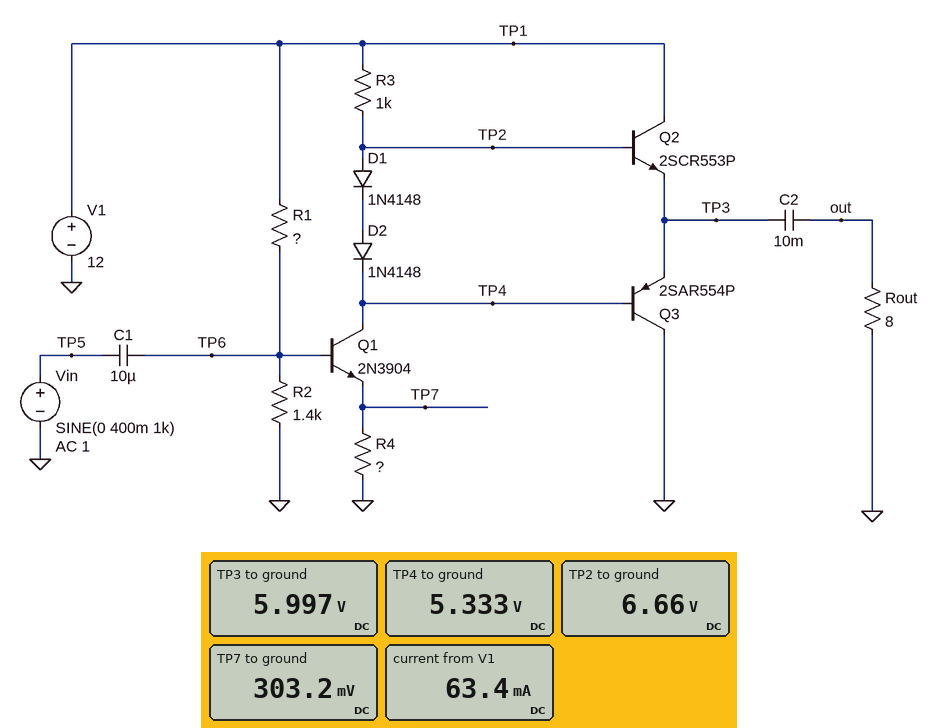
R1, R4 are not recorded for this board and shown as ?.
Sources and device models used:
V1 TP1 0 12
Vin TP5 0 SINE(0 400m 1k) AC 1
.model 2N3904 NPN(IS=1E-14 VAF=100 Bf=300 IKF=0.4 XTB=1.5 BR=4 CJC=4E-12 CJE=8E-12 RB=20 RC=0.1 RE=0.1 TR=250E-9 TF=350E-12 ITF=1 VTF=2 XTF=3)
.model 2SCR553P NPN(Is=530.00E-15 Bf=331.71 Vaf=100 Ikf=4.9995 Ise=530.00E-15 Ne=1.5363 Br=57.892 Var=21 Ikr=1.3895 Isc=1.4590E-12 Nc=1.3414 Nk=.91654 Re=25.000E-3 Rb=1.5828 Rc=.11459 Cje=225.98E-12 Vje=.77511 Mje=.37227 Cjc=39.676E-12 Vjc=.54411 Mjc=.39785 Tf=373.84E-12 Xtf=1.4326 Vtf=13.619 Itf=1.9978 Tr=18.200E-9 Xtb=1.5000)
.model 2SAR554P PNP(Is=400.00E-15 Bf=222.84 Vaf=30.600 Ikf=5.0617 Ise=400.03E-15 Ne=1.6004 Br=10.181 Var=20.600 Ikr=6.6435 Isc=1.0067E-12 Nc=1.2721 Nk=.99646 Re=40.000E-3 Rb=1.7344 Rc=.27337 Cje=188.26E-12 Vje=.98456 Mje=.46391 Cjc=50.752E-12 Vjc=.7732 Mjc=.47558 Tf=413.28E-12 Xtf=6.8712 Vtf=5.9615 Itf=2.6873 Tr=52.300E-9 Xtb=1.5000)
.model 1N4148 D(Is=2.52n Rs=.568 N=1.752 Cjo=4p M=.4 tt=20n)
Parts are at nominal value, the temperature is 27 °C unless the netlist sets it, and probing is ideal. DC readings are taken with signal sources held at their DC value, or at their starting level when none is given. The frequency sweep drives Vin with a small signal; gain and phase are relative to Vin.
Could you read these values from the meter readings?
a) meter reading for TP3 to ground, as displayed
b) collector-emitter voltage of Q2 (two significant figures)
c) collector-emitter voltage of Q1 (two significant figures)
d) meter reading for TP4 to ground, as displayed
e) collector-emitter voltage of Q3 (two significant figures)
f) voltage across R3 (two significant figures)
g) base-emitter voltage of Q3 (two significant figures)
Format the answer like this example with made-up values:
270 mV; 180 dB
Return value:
5.997 V; 6.0 V; 5.0 V; 5.333 V; -6.0 V; 5.3 V; -660 mV
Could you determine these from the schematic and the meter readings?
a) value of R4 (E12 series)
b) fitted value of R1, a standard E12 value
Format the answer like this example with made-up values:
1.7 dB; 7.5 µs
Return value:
56 Ω; 15 kΩ
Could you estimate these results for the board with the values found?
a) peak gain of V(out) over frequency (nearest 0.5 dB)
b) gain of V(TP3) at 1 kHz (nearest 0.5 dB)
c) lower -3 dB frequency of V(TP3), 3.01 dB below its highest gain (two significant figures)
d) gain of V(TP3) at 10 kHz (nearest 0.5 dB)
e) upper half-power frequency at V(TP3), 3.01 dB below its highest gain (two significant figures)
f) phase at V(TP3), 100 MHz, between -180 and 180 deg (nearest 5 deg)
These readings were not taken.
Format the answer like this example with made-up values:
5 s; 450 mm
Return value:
20.5 dB; 20.5 dB; 13 Hz; 20.5 dB; 2.2 MHz; 80 deg
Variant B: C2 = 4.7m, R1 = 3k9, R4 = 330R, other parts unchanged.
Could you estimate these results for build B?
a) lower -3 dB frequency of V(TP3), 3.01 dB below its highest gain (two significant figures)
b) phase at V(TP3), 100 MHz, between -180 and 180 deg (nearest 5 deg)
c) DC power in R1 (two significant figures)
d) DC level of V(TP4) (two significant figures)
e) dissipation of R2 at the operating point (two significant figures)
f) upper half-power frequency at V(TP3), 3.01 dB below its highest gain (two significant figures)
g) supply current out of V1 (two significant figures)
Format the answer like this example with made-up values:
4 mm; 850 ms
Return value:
15 Hz; 50 deg; 20 mW; 3.4 V; 7.1 mW; 2.3 MHz; 100 mA
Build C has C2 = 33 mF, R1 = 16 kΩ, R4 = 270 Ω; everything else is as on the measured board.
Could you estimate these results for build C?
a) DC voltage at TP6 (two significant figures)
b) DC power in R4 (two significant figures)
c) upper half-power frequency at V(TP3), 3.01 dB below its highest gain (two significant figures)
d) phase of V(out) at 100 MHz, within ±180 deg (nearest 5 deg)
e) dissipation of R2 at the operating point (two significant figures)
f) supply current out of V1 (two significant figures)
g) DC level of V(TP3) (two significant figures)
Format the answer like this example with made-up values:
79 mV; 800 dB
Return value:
960 mV; 340 µW; 800 kHz; 95 deg; 660 µW; 5.9 mA; 10 V
